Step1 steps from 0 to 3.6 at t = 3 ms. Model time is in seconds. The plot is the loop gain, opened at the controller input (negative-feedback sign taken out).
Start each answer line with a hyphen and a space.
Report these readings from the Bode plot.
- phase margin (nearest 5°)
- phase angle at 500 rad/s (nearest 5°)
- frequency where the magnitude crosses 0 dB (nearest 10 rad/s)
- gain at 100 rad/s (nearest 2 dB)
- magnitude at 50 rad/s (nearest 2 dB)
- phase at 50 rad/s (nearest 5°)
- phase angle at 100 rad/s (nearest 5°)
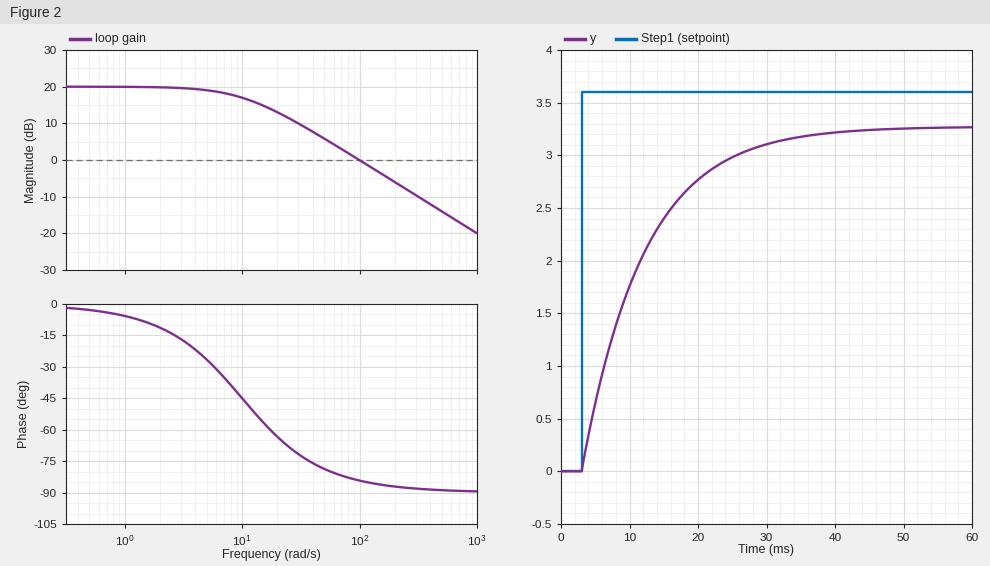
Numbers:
- 95°
- -90°
- 100 rad/s
- 0 dB
- 6 dB
- -80°
- -85°
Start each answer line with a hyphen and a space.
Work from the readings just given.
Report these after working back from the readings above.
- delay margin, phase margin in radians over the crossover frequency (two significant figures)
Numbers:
- 0.017 s
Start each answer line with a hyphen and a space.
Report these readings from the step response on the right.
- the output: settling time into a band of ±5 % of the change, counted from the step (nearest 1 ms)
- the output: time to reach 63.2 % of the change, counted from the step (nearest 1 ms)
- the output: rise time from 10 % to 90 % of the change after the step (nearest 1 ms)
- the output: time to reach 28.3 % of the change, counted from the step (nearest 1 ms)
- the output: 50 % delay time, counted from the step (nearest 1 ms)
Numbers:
- 27 ms
- 9 ms
- 20 ms
- 3 ms
- 6 ms
